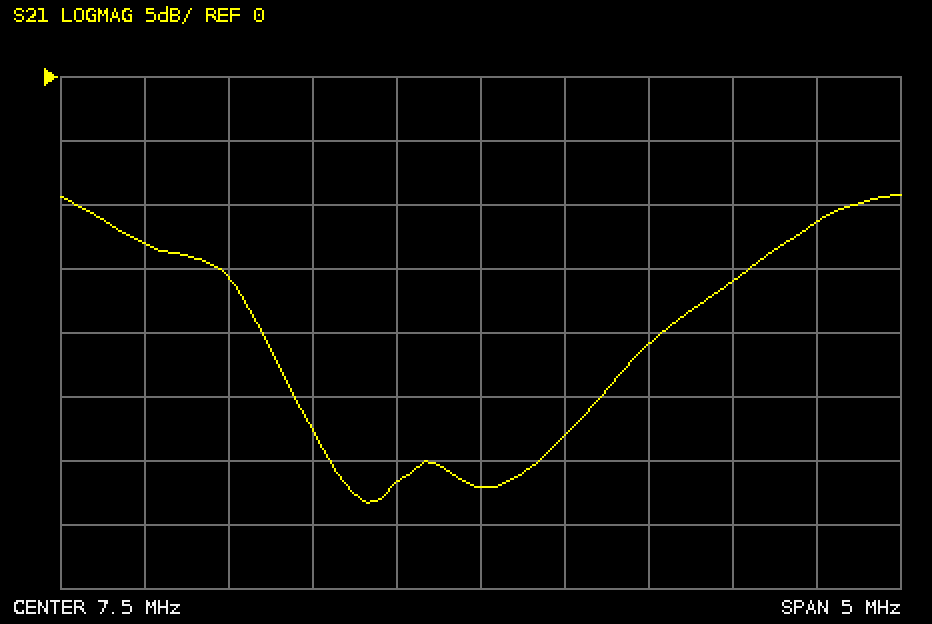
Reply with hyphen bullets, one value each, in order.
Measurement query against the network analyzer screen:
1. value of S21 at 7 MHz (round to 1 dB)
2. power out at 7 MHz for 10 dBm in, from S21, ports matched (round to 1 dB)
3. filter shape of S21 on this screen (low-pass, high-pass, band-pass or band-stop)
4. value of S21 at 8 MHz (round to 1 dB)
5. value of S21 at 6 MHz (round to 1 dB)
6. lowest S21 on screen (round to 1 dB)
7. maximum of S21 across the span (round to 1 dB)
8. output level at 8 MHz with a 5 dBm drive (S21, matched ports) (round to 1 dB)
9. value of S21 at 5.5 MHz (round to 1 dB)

- -32 dB
- -22 dBm
- band-stop
- -28 dB
- -16 dB
- -33 dB
- -9 dB
- -23 dBm
- -13 dB
